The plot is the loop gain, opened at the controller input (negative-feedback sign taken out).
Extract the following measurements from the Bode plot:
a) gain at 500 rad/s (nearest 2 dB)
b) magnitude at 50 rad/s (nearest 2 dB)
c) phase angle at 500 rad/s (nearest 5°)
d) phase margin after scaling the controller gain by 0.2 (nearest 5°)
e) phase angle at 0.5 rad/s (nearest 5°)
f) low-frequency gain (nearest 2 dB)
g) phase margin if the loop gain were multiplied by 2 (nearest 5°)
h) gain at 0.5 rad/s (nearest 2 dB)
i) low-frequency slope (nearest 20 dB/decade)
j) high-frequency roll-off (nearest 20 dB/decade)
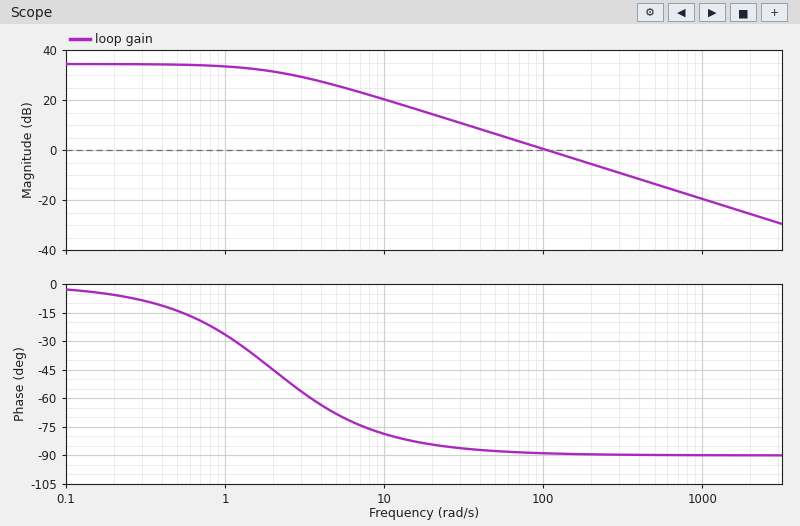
-14 dB
6 dB
-90°
95°
-15°
34 dB
90°
34 dB
0 dB/decade
-20 dB/decade
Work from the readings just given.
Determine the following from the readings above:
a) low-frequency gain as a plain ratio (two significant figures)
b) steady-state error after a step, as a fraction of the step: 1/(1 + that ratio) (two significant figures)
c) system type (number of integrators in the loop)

50
0.020
0
